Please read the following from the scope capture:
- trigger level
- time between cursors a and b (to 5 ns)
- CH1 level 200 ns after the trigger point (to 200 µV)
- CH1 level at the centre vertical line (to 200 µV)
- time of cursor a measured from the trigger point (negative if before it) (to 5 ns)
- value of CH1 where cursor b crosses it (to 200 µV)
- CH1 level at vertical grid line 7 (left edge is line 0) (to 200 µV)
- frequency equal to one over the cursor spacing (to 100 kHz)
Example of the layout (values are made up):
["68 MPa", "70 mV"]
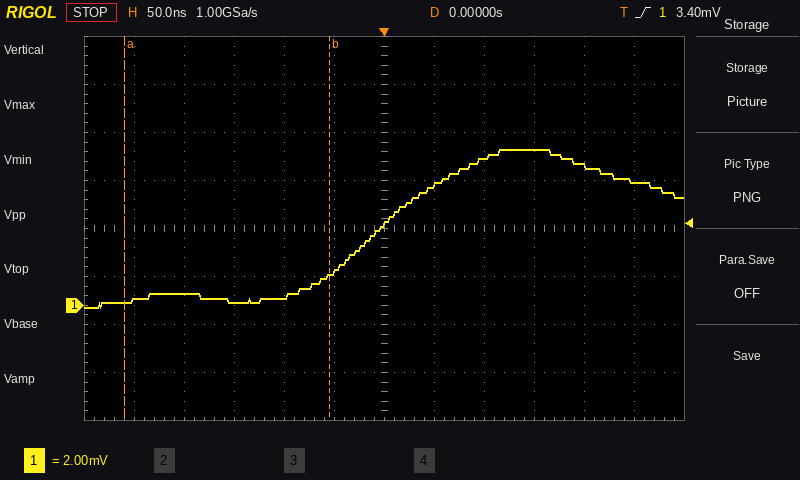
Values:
["3.40 mV", "205 ns", "5.8 mV", "3.4 mV", "-260 ns", "1.2 mV", "5.0 mV", "4.9 MHz"]
